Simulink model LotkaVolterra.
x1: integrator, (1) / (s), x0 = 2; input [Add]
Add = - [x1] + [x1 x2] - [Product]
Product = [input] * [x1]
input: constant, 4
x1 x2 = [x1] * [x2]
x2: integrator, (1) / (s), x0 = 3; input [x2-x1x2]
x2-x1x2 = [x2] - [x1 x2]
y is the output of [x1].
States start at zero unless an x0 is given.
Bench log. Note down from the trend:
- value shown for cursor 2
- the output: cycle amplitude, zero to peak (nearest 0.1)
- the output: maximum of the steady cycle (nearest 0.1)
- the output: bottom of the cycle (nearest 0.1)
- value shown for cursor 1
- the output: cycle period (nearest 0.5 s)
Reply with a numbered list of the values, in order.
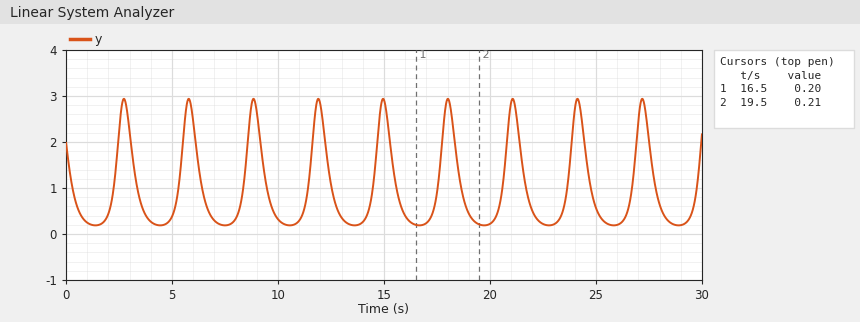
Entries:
1. 0.21
2. 1.4
3. 2.9
4. 0.2
5. 0.20
6. 3.0 s
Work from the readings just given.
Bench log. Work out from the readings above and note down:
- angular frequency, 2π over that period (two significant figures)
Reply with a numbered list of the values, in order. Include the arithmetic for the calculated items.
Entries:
1. 2π / 3 = 2.1 rad/s
